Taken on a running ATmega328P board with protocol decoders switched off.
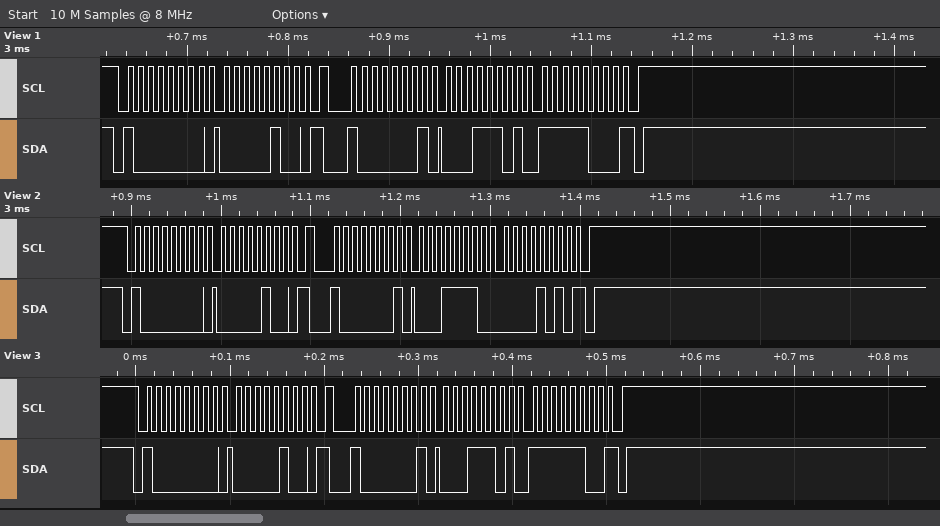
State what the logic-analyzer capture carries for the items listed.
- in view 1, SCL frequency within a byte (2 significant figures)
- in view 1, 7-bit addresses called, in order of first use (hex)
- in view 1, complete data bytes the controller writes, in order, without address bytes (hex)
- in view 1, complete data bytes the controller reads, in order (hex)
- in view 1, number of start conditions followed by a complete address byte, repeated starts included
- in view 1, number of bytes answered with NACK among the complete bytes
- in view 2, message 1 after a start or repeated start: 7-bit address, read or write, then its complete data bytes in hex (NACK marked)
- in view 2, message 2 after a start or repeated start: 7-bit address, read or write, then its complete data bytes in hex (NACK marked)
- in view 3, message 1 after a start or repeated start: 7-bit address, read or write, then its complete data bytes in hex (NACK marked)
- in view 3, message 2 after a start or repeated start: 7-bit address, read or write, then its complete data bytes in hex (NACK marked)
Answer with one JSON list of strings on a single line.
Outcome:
["100 kHz", "0x40", "04", "1D F8", "2", "1", "0x40 write: 04", "0x40 read: 1E 0A NACK", "0x40 write: 04", "0x40 read: 1D FC NACK"]
